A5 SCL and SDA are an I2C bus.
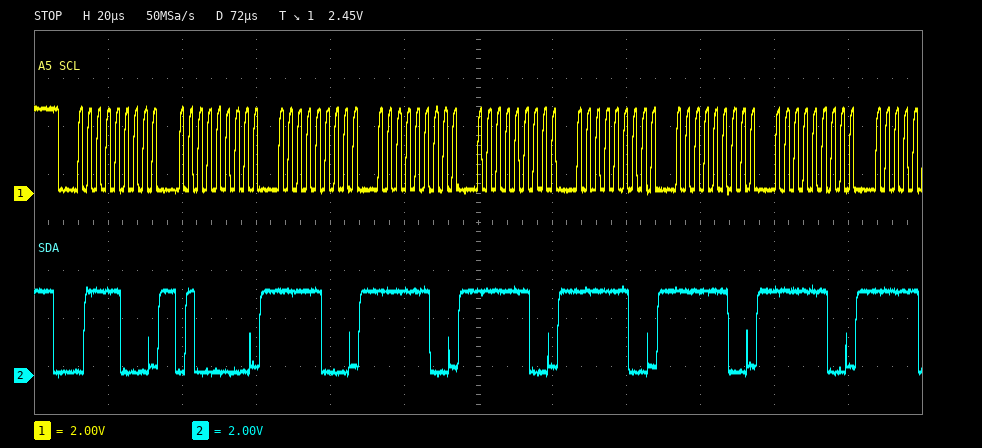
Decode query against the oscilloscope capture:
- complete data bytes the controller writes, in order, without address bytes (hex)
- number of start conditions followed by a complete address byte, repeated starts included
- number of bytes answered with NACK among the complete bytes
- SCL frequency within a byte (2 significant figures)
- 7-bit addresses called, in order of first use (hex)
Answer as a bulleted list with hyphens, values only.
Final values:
- 40 F8 FC FC FC FC FC
- 1
- 0
- 400 kHz
- 0x3C
